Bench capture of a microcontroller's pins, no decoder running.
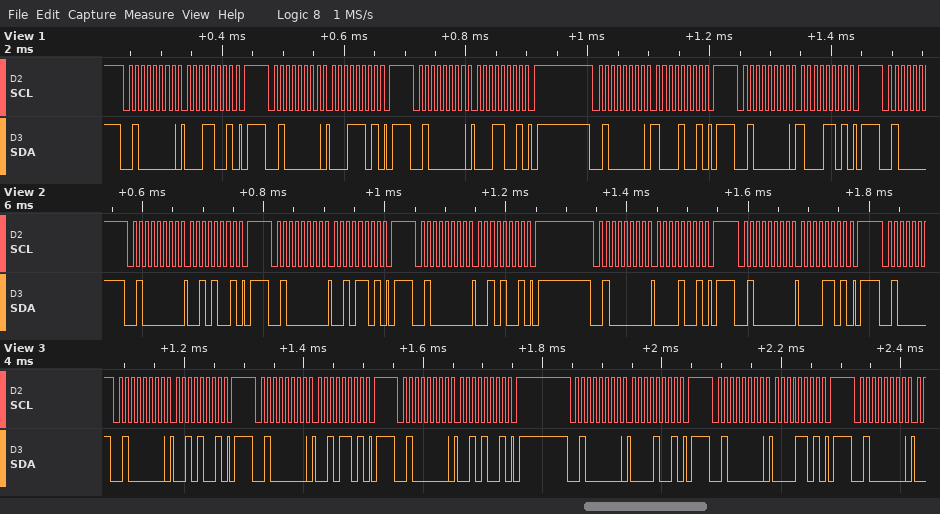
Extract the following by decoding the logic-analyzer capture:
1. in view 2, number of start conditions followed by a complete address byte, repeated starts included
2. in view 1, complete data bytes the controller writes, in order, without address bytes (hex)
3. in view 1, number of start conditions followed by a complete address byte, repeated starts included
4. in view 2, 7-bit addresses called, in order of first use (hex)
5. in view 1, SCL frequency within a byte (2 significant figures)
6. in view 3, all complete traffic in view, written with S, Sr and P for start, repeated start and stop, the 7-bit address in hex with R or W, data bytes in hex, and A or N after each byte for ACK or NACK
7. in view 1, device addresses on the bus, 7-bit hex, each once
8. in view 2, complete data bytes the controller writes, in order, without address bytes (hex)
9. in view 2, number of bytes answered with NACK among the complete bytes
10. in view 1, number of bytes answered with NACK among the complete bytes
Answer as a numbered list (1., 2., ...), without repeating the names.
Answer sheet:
1. 5
2. 19 1D 19 89 8D
3. 5
4. 0x20
5. 100 kHz
6. S 20W A 29 A P S 20W A 2D A P S 20W A 29 A P S 20W A 09 A P S 20W A 0D A P S 20W A
7. 0x20
8. 29 2D 29 09 0D
9. 0
10. 0
